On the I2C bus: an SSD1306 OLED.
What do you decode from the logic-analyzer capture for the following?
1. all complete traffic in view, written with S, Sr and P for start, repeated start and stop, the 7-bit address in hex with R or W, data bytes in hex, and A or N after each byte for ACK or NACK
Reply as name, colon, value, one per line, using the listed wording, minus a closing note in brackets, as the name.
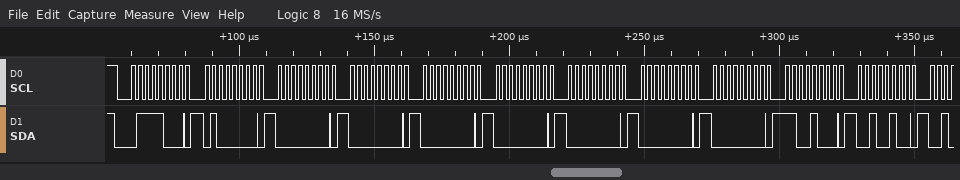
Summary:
all complete traffic in view, written with S, Sr and P for start, repeated start and stop, the 7-bit address in hex with R or W, data bytes in hex, and A or N after each byte for ACK or NACK: S 3CW A 40 A 00 A 00 A 00 A 00 A 00 A 00 A 00 A C8 A 24 A
